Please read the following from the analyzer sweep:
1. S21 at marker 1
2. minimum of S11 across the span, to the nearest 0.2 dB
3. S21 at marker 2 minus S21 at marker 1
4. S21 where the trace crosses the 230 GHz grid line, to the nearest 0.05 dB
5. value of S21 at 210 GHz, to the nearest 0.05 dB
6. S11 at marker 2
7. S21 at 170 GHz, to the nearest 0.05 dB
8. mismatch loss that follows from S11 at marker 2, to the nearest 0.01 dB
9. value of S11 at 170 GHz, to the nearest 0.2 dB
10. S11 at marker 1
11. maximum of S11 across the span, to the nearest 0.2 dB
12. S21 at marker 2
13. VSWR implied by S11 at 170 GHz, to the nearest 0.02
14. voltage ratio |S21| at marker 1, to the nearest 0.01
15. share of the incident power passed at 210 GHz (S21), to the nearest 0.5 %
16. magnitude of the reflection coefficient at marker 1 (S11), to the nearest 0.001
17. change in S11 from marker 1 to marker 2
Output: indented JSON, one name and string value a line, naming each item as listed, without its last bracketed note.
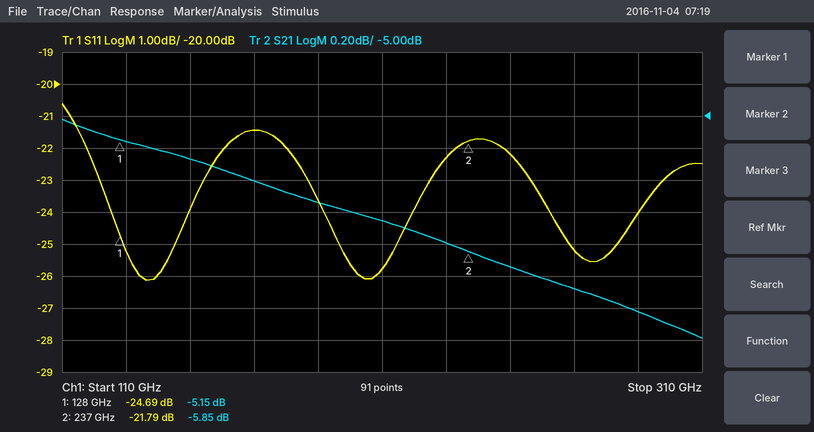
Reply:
{
  "S21 at marker 1": "-5.15 dB",
  "minimum of S11 across the span, to the nearest 0.2 dB": "-26.2 dB",
  "S21 at marker 2 minus S21 at marker 1": "-0.70 dB",
  "S21 where the trace crosses the 230 GHz grid line, to the nearest 0.05 dB": "-5.80 dB",
  "value of S21 at 210 GHz, to the nearest 0.05 dB": "-5.65 dB",
  "S11 at marker 2": "-21.79 dB",
  "S21 at 170 GHz, to the nearest 0.05 dB": "-5.40 dB",
  "mismatch loss that follows from S11 at marker 2, to the nearest 0.01 dB": "0.03 dB",
  "value of S11 at 170 GHz, to the nearest 0.2 dB": "-21.4 dB",
  "S11 at marker 1": "-24.69 dB",
  "maximum of S11 across the span, to the nearest 0.2 dB": "-20.6 dB",
  "S21 at marker 2": "-5.85 dB",
  "VSWR implied by S11 at 170 GHz, to the nearest 0.02": "1.18",
  "voltage ratio |S21| at marker 1, to the nearest 0.01": "0.55",
  "share of the incident power passed at 210 GHz (S21), to the nearest 0.5 %": "27.0 %",
  "magnitude of the reflection coefficient at marker 1 (S11), to the nearest 0.001": "0.058",
  "change in S11 from marker 1 to marker 2": "2.90 dB"
}
